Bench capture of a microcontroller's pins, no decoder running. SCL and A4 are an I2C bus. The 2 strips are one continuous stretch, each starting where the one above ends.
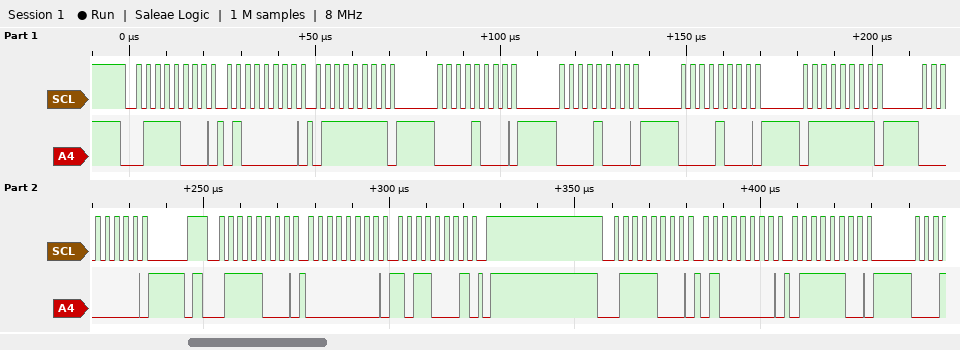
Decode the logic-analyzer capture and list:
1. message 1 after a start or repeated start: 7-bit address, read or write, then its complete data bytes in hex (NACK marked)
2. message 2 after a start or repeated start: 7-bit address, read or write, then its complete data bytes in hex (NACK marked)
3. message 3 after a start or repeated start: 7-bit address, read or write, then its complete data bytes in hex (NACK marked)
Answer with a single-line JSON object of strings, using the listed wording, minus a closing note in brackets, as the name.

{"message 1 after a start or repeated start: 7-bit address, read or write, then its complete data bytes in hex": "0x3C write: 40 7F 08 08 08 7F 00", "message 2 after a start or repeated start: 7-bit address, read or write, then its complete data bytes in hex": "0x3C write: 00 B1", "message 3 after a start or repeated start: 7-bit address, read or write, then its complete data bytes in hex": "0x3C write: 40 7C"}
